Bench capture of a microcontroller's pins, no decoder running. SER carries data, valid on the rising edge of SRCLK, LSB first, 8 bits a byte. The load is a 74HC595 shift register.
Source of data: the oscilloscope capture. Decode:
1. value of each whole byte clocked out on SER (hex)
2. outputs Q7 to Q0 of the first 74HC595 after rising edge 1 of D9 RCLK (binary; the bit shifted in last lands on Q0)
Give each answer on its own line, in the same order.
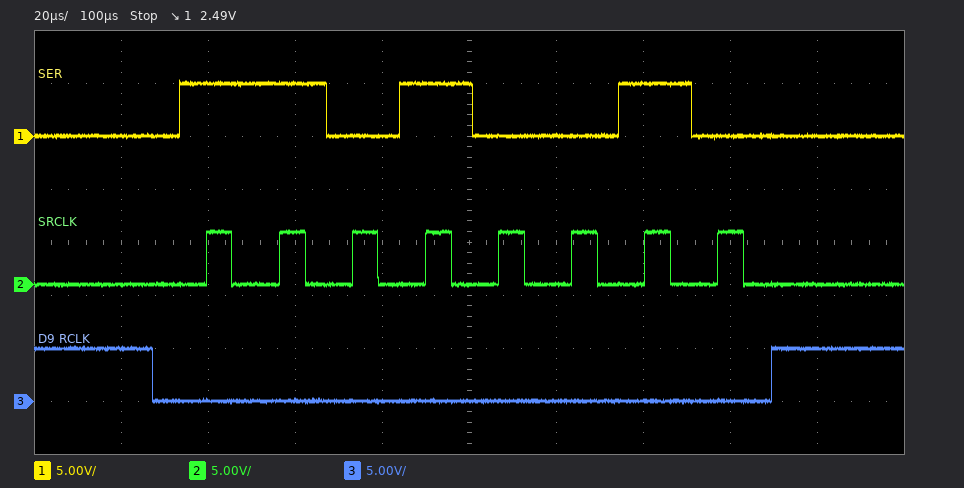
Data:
4B
11010010
